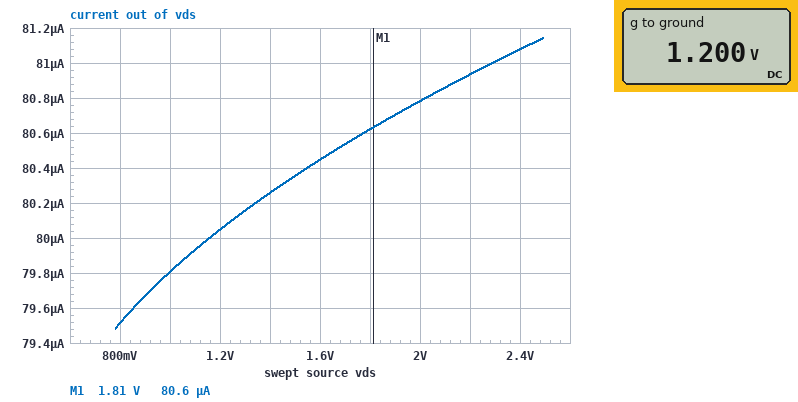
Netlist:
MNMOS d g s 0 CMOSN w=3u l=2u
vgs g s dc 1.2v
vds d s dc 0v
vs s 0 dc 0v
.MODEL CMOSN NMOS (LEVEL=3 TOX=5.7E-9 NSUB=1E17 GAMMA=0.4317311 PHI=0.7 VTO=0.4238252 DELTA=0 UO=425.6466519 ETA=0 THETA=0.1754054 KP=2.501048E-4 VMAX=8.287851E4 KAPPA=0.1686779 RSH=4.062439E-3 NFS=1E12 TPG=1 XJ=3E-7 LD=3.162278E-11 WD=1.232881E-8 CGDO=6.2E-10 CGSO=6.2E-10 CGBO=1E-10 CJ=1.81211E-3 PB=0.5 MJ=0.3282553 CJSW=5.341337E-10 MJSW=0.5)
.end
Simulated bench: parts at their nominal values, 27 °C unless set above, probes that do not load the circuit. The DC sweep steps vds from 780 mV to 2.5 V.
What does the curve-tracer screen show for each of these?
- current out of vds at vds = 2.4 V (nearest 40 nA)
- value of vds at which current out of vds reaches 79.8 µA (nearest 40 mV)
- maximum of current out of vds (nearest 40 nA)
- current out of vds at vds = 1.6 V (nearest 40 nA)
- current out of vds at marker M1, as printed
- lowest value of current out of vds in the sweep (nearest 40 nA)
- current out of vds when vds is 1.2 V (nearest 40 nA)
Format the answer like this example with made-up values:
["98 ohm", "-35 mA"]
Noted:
["81.08 µA", "1.00 V", "81.16 µA", "80.44 µA", "80.6 µA", "79.48 µA", "80.04 µA"]
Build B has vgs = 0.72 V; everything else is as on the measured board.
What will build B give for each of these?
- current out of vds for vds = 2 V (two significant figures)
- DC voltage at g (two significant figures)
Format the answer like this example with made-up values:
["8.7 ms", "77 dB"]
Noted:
["15 µA", "720 mV"]
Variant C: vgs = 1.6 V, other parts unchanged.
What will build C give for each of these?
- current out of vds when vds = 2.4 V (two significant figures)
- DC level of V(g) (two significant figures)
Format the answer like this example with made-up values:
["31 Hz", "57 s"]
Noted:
["160 µA", "1.6 V"]
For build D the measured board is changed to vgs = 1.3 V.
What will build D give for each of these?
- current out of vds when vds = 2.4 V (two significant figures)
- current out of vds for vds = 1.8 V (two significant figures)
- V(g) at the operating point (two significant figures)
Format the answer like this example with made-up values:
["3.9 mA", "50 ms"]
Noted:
["100 µA", "99 µA", "1.3 V"]
